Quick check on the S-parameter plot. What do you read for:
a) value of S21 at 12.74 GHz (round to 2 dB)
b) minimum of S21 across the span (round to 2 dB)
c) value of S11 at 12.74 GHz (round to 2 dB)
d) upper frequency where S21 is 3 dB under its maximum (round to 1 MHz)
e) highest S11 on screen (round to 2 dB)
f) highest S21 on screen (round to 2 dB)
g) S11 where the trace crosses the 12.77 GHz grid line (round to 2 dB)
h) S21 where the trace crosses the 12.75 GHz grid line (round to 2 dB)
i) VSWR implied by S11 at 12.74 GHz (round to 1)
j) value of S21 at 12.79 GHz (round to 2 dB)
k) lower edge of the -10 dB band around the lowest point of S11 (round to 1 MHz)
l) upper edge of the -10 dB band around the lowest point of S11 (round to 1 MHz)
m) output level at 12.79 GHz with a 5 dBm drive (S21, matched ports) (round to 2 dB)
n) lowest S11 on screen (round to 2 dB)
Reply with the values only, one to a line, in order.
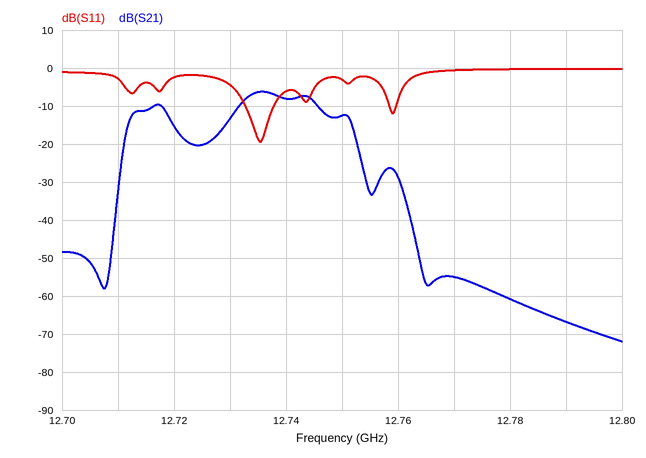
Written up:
-8 dB
-72 dB
-6 dB
12.745 GHz
0 dB
-6 dB
0 dB
-12 dB
3
-66 dB
12.733 GHz
12.738 GHz
-62 dBm
-20 dB
